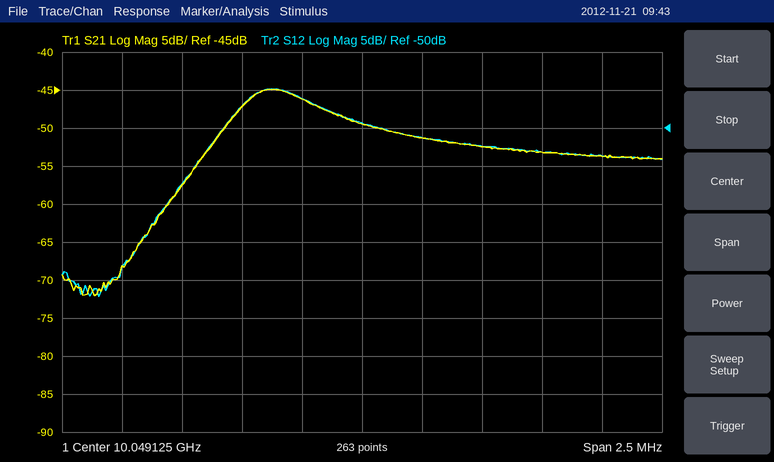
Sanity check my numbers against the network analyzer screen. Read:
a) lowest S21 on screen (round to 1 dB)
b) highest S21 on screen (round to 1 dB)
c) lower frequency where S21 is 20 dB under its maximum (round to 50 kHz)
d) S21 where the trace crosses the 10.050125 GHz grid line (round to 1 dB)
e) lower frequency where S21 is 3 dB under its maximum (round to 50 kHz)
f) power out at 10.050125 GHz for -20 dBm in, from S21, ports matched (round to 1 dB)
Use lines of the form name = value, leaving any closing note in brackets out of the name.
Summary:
lowest S21 on screen = -72 dB
highest S21 on screen = -45 dB
lower frequency where S21 is 20 dB under its maximum = 10.04820 GHz
S21 where the trace crosses the 10.050125 GHz grid line = -54 dB
lower frequency where S21 is 3 dB under its maximum = 10.04860 GHz
power out at 10.050125 GHz for -20 dBm in, from S21, ports matched = -74 dBm
